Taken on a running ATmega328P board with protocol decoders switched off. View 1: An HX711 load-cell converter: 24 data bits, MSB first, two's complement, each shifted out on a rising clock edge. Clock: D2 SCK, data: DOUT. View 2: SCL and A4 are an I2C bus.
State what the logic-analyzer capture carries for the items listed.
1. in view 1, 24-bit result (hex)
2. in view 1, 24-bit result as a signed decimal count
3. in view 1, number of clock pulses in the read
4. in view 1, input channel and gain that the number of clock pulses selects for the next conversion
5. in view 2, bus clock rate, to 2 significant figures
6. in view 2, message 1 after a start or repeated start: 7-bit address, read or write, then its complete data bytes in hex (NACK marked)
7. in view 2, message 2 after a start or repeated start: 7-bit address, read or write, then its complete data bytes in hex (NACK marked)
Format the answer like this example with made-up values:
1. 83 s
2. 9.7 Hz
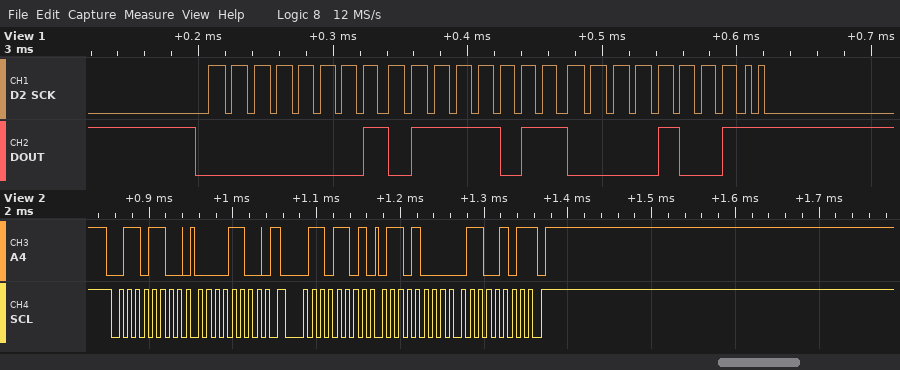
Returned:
1. 0x017B09
2. 97033
3. 26
4. channel B, gain 32
5. 100 kHz
6. 0x36 write: 0C
7. 0x36 read: 68 65 NACK
